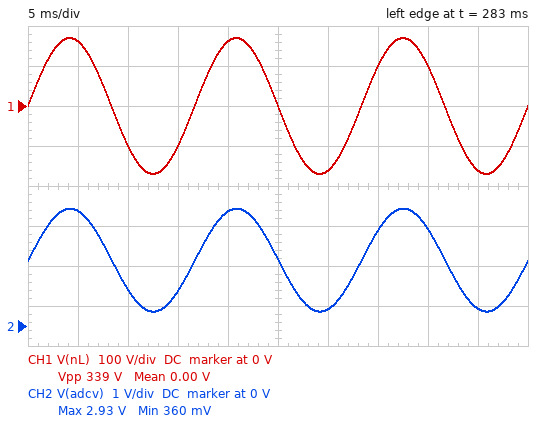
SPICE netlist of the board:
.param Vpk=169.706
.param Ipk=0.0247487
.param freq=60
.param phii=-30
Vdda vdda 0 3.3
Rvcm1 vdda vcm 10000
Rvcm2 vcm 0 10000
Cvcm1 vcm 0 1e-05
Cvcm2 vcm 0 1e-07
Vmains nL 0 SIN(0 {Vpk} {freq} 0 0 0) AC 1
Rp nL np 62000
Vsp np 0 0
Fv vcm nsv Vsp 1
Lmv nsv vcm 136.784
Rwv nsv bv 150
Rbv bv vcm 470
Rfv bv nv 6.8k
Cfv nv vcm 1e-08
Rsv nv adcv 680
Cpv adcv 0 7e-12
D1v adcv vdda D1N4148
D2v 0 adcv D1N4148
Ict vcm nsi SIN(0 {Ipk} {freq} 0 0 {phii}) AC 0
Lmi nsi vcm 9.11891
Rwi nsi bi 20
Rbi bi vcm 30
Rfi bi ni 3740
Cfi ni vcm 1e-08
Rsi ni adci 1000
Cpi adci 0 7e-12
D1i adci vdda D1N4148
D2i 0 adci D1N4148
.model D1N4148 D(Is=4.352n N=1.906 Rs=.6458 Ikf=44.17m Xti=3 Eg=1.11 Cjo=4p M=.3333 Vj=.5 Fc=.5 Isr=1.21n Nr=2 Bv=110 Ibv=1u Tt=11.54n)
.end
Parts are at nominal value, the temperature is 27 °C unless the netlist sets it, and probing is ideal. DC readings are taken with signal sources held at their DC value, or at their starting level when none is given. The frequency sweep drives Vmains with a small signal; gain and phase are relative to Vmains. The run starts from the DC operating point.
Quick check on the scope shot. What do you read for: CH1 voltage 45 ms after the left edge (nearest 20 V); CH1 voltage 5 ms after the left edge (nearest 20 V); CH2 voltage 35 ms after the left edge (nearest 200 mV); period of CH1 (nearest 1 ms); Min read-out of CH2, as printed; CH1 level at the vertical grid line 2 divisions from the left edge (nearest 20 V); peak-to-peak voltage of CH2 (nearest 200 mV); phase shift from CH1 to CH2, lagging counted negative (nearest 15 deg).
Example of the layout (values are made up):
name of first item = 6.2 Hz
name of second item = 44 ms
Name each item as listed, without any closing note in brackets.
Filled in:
CH1 voltage 45 ms after the left edge = -160 V
CH1 voltage 5 ms after the left edge = 160 V
CH2 voltage 35 ms after the left edge = 2.4 V
period of CH1 = 17 ms
Min read-out of CH2, as printed = 360 mV
CH1 level at the vertical grid line 2 divisions from the left edge = -100 V
peak-to-peak voltage of CH2 = 2.6 V
phase shift from CH1 to CH2, lagging counted negative = 0 deg
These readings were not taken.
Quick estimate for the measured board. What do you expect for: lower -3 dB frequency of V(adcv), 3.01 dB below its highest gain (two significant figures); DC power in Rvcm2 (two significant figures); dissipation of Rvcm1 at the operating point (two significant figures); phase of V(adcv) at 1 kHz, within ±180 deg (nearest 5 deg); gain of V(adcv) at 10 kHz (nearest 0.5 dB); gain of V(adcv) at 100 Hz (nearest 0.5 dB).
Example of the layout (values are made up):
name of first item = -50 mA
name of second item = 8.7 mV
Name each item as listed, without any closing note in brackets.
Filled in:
lower -3 dB frequency of V(adcv), 3.01 dB below its highest gain = 720 mHz
DC power in Rvcm2 = 270 µW
dissipation of Rvcm1 at the operating point = 270 µW
phase of V(adcv) at 1 kHz, within ±180 deg = -25 deg
gain of V(adcv) at 10 kHz = -56.0 dB
gain of V(adcv) at 100 Hz = -42.5 dB
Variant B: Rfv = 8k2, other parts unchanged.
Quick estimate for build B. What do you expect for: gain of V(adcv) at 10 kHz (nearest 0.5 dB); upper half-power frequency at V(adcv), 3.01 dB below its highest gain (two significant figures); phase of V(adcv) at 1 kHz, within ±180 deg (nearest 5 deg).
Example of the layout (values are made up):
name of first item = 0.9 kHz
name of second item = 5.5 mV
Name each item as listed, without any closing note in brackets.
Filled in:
gain of V(adcv) at 10 kHz = -57.5 dB
upper half-power frequency at V(adcv), 3.01 dB below its highest gain = 1.8 kHz
phase of V(adcv) at 1 kHz, within ±180 deg = -30 deg
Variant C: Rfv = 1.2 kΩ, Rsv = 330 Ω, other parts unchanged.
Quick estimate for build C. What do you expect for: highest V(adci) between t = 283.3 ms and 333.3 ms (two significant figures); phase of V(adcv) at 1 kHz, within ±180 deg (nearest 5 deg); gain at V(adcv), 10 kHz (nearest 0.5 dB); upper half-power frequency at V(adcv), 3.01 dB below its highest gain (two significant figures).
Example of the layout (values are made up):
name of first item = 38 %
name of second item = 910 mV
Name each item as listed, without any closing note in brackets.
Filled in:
highest V(adci) between t = 283.3 ms and 333.3 ms = 2.5 V
phase of V(adcv) at 1 kHz, within ±180 deg = -5 deg
gain at V(adcv), 10 kHz = -45.5 dB
upper half-power frequency at V(adcv), 3.01 dB below its highest gain = 9.5 kHz
